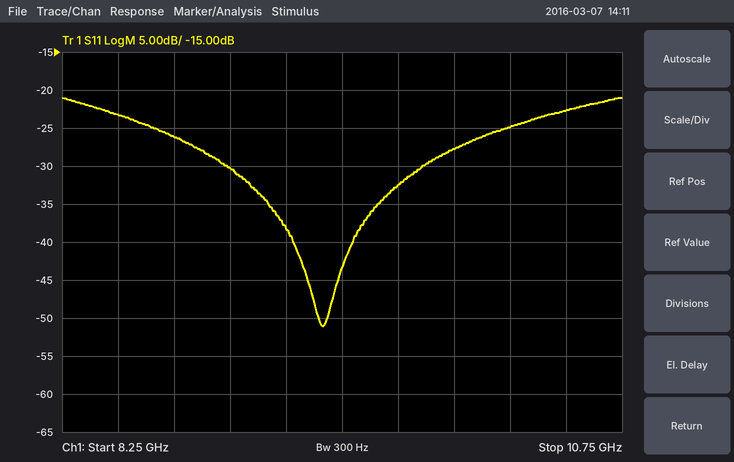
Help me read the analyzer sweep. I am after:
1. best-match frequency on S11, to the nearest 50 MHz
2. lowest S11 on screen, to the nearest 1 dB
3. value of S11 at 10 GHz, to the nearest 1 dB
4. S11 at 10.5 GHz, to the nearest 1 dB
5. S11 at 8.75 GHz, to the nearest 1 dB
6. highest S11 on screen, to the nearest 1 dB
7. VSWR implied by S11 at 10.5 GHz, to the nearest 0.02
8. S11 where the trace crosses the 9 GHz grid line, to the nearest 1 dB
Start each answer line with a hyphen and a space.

- 9.40 GHz
- -51 dB
- -28 dB
- -23 dB
- -26 dB
- -21 dB
- 1.16
- -30 dB
